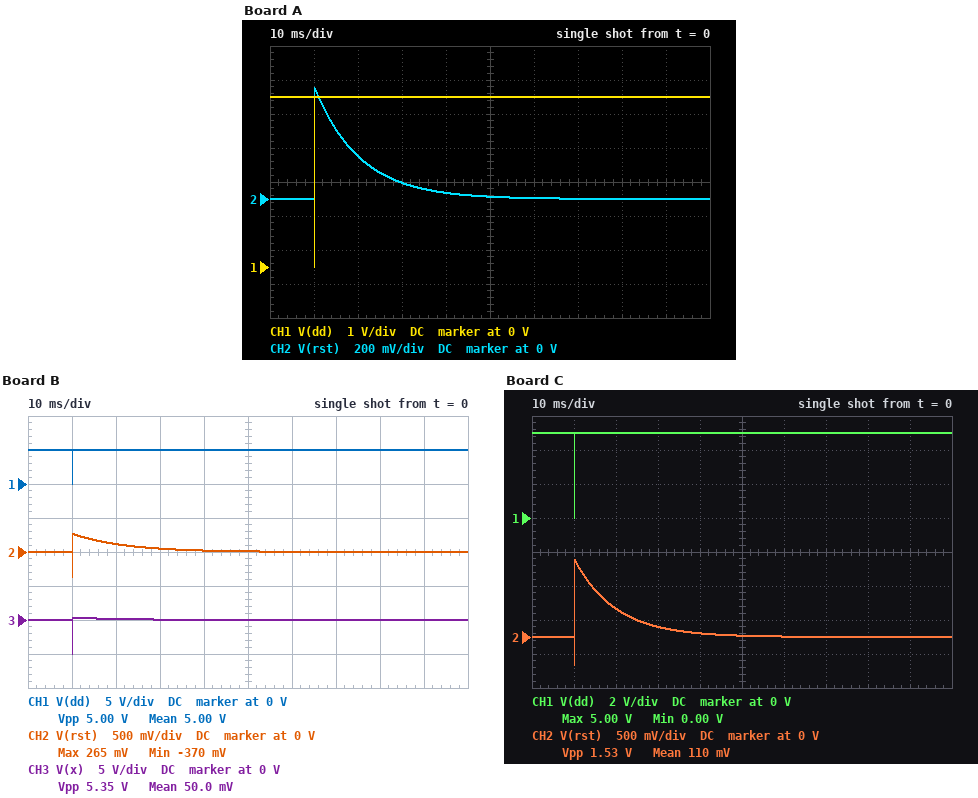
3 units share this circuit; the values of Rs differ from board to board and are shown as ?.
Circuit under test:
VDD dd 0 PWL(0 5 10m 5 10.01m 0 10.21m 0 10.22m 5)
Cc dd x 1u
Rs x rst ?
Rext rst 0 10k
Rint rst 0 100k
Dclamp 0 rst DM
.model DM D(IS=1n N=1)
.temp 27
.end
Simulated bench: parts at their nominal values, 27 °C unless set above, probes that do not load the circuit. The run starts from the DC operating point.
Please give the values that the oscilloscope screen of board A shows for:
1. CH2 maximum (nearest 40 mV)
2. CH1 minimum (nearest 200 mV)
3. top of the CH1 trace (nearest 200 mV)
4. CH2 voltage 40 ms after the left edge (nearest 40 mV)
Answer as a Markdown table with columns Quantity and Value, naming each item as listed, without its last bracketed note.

| Quantity | Value |
|---|---|
| CH2 maximum | 640 mV |
| CH1 minimum | 0 V |
| top of the CH1 trace | 5.0 V |
| CH2 voltage 40 ms after the left edge | 40 mV |
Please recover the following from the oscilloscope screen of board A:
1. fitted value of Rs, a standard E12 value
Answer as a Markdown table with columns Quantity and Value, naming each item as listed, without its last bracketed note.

| Quantity | Value |
|---|---|
| fitted value of Rs, a standard E12 value | 1.2 kΩ |
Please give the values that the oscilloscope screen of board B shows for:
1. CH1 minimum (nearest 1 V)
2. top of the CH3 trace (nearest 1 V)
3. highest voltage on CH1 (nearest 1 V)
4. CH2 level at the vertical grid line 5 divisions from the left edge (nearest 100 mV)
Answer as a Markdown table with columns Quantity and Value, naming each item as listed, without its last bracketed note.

| Quantity | Value |
|---|---|
| CH1 minimum | 0 V |
| top of the CH3 trace | 0 V |
| highest voltage on CH1 | 5 V |
| CH2 level at the vertical grid line 5 divisions from the left edge | 0 V |
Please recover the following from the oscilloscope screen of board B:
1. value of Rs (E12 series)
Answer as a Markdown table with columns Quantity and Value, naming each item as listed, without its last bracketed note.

| Quantity | Value |
|---|---|
| value of Rs | 2.7 kΩ |
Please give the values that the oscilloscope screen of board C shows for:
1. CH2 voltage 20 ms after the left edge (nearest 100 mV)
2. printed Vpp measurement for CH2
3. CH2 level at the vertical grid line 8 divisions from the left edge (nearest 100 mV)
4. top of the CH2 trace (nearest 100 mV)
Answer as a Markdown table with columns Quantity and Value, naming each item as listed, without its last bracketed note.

| Quantity | Value |
|---|---|
| CH2 voltage 20 ms after the left edge | 400 mV |
| printed Vpp measurement for CH2 | 1.53 V |
| CH2 level at the vertical grid line 8 divisions from the left edge | 0 V |
| top of the CH2 trace | 1.1 V |
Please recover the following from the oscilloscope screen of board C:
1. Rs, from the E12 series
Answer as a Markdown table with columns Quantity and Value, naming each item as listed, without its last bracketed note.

| Quantity | Value |
|---|---|
| Rs, from the E12 series | 680 Ω |
